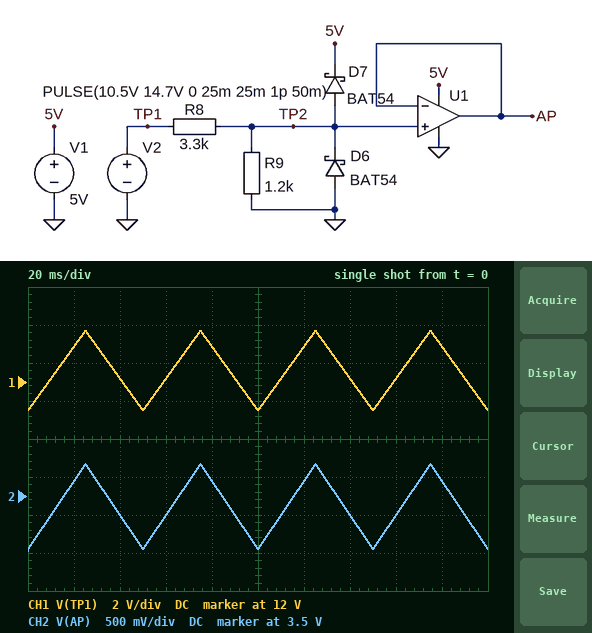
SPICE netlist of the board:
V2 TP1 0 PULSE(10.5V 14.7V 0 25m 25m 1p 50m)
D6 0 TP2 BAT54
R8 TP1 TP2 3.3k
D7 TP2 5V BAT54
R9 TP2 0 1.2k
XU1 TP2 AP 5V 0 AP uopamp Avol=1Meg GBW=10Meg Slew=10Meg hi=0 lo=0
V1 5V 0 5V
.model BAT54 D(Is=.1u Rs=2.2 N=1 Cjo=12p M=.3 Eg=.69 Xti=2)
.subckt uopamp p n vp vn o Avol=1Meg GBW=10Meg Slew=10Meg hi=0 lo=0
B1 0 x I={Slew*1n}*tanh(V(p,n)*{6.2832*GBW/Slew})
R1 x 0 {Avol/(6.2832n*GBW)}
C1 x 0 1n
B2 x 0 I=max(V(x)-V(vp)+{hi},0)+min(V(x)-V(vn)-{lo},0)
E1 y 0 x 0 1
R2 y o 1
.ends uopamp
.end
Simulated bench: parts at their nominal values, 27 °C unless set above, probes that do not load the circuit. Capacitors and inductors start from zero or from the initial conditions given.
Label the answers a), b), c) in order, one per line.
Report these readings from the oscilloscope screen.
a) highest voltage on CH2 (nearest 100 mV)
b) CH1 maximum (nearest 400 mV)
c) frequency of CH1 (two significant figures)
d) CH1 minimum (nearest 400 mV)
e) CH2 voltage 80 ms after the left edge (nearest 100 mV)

a) 3.9 V
b) 14.8 V
c) 20 Hz
d) 10.4 V
e) 3.7 V
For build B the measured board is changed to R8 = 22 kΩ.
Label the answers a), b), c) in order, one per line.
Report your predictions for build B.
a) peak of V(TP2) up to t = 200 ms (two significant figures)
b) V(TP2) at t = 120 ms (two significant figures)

a) 760 mV
b) 720 mV
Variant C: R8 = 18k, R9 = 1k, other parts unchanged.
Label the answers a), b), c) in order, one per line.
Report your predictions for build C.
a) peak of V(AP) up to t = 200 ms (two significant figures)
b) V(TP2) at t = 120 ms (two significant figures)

a) 770 mV
b) 730 mV
